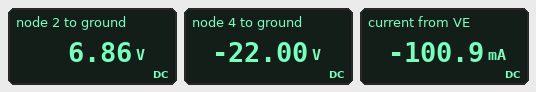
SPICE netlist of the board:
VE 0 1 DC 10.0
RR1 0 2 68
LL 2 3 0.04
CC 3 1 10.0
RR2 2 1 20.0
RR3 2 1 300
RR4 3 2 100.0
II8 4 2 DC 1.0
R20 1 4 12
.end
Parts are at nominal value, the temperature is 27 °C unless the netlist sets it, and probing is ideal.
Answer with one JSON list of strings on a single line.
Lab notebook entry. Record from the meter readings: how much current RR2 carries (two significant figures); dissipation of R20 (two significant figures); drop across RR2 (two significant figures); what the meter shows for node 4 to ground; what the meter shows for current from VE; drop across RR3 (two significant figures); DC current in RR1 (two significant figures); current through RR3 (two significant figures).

["840 mA", "12 W", "17 V", "-22.00 V", "-100.9 mA", "17 V", "100 mA", "56 mA"]
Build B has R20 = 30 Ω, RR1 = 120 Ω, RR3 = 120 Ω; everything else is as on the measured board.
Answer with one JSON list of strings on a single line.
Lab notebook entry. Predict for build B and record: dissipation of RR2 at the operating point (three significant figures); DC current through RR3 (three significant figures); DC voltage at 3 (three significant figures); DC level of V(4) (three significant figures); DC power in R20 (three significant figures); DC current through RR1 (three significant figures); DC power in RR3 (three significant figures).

["13.2 W", "135 mA", "6.25 V", "-40.0 V", "30.0 W", "52.1 mA", "2.20 W"]
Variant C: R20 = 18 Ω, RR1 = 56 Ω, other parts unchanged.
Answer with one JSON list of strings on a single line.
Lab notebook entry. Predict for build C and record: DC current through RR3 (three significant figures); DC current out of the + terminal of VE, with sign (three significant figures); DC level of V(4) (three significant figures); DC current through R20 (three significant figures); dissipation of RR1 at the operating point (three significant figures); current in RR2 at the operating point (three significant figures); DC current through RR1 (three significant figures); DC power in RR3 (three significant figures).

["55.2 mA", "-117 mA", "-28.0 V", "1.00 A", "767 mW", "828 mA", "117 mA", "914 mW"]
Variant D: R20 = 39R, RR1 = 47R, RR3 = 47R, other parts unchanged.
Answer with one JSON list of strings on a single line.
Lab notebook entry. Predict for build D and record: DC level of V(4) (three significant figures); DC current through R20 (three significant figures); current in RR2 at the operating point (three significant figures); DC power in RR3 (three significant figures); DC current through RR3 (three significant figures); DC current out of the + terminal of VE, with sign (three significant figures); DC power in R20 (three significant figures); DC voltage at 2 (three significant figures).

["-49.0 V", "1.00 A", "655 mA", "3.65 W", "279 mA", "-66.0 mA", "39.0 W", "3.10 V"]
